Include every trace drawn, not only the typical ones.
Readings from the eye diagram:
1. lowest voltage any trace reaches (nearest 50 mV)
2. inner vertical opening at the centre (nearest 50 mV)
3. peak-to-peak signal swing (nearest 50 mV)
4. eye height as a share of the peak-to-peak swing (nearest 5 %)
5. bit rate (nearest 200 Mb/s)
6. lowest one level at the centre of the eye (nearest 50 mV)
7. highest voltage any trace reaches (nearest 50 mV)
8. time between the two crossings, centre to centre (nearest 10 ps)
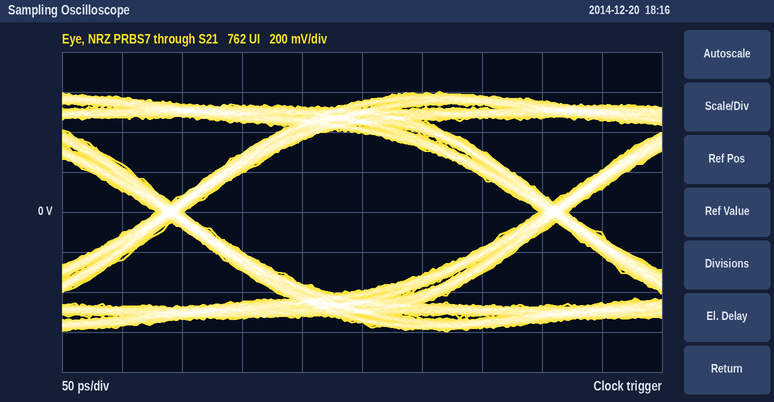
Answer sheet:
-600 mV
800 mV
1.20 V
65 %
3.2 Gb/s
400 mV
600 mV
320 ps
